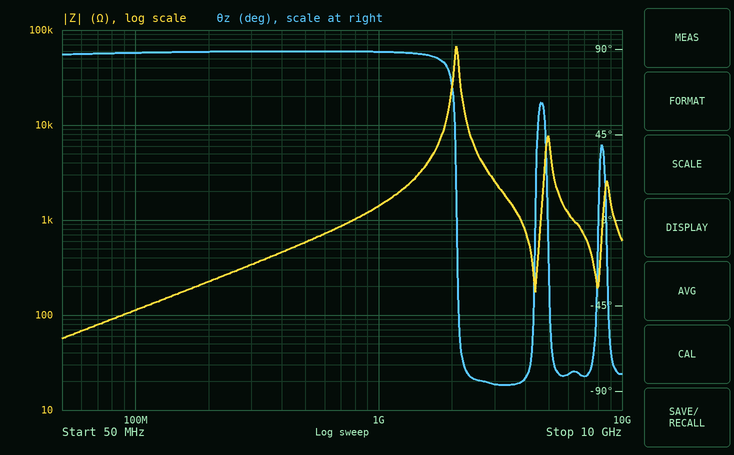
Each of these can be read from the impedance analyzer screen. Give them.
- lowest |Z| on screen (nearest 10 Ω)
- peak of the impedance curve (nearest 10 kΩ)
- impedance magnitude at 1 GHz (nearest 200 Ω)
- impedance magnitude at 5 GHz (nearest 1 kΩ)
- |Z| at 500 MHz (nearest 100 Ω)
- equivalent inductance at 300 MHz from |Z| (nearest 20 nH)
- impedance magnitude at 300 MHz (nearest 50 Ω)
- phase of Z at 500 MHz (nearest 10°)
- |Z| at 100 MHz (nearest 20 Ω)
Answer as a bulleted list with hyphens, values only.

- 60 Ω
- 70 kΩ
- 1.4 kΩ
- 7 kΩ
- 600 Ω
- 180 nH
- 350 Ω
- 90°
- 120 Ω
